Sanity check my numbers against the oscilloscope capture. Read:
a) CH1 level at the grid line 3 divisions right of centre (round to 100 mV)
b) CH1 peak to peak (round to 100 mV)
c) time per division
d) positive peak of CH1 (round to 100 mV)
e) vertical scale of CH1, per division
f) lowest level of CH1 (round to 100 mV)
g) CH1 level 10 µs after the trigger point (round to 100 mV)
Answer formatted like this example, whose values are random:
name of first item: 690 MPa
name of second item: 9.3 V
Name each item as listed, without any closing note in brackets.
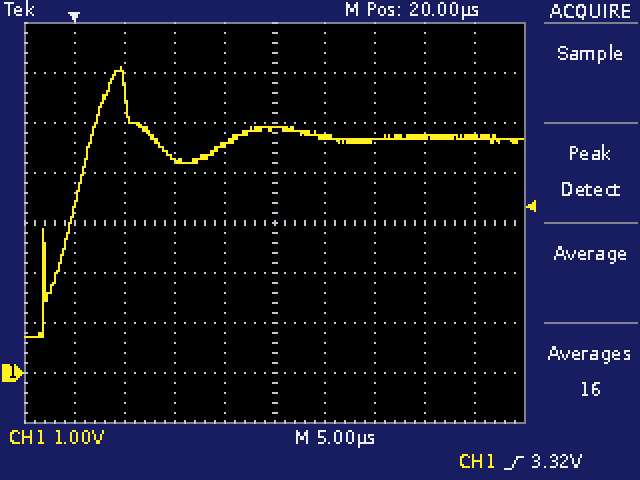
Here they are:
CH1 level at the grid line 3 divisions right of centre: 4.7 V
CH1 peak to peak: 5.4 V
time per division: 5 µs
positive peak of CH1: 6.1 V
vertical scale of CH1, per division: 1 V
lowest level of CH1: 700 mV
CH1 level 10 µs after the trigger point: 4.3 V
